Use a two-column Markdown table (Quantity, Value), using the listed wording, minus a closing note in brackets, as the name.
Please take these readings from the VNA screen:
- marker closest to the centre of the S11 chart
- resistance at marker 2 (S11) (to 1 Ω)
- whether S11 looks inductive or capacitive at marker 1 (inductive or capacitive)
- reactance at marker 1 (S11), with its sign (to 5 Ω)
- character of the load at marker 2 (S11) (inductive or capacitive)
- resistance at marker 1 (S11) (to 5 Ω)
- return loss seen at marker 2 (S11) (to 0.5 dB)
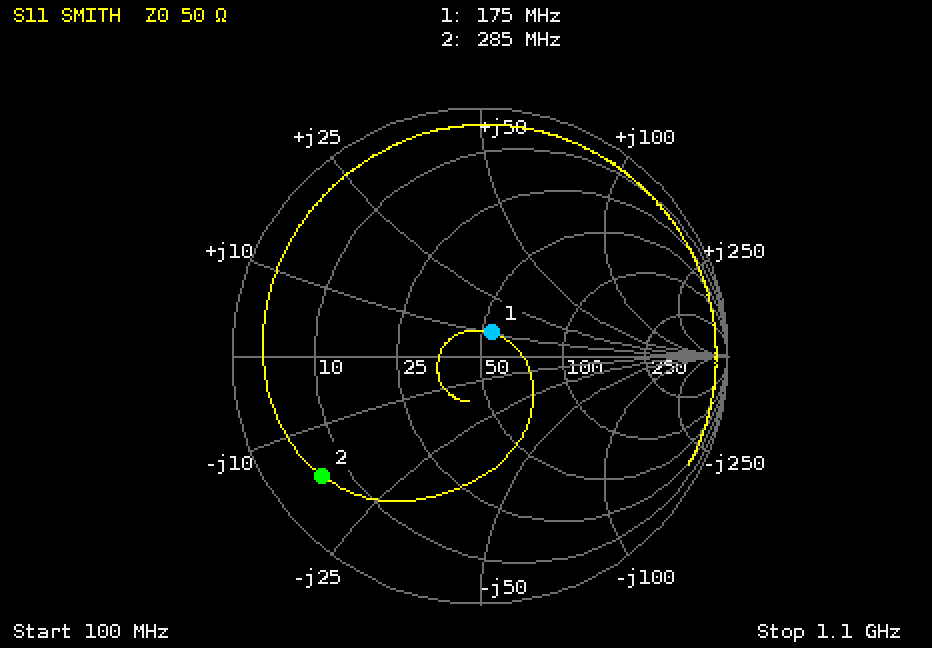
| Quantity | Value |
|---|---|
| marker closest to the centre of the S11 chart | marker 1 |
| resistance at marker 2 (S11) | 6 Ω |
| whether S11 looks inductive or capacitive at marker 1 | inductive |
| reactance at marker 1 (S11), with its sign | +10 Ω |
| character of the load at marker 2 (S11) | capacitive |
| resistance at marker 1 (S11) | 55 Ω |
| return loss seen at marker 2 (S11) | 2.0 dB |
